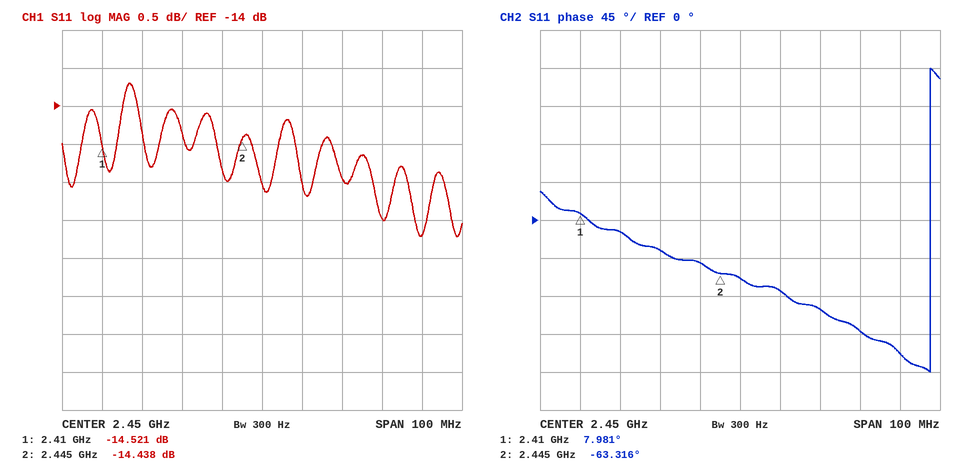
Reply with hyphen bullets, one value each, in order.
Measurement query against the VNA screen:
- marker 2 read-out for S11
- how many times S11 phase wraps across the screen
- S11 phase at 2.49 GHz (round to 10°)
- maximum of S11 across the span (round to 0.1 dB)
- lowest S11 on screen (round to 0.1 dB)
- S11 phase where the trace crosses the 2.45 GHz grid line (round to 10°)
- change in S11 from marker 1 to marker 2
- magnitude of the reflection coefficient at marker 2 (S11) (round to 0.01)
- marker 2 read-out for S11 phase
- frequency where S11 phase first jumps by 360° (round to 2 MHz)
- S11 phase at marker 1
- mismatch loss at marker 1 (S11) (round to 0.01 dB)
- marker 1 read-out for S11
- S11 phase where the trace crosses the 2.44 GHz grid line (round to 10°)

- -14.438 dB
- 1
- -160°
- -13.7 dB
- -15.7 dB
- -70°
- 0.083 dB
- 0.19
- -63.316°
- 2.498 GHz
- 7.981°
- 0.16 dB
- -14.521 dB
- -50°
